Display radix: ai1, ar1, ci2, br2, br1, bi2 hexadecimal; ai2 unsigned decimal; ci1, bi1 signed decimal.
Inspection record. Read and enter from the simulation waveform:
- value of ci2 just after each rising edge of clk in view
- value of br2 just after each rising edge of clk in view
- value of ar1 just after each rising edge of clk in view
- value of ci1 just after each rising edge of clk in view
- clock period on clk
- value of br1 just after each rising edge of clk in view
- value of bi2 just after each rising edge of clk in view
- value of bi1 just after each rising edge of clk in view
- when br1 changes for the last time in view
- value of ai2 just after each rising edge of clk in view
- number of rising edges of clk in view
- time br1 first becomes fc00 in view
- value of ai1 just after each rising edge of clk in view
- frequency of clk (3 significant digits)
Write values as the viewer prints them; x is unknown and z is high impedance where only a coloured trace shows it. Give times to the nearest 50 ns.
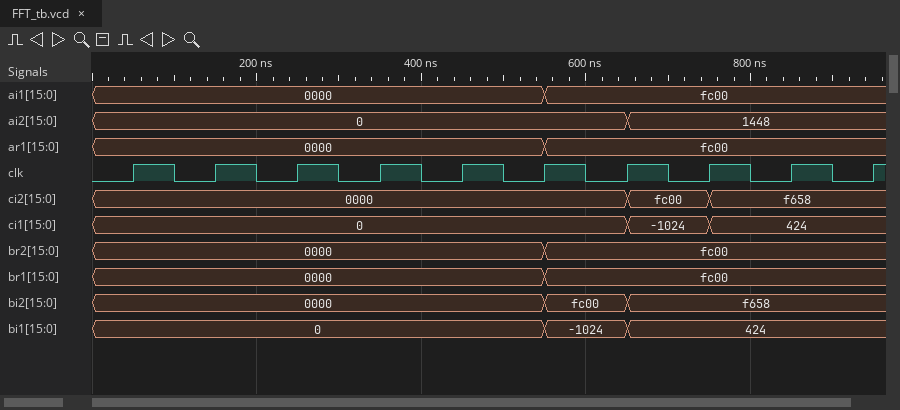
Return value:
0000, 0000, 0000, 0000, 0000, 0000, fc00, f658, f658, f658
0000, 0000, 0000, 0000, 0000, fc00, fc00, fc00, fc00, fc00
0000, 0000, 0000, 0000, 0000, fc00, fc00, fc00, fc00, fc00
0, 0, 0, 0, 0, 0, -1024, 424, 424, 424
100 ns
0000, 0000, 0000, 0000, 0000, fc00, fc00, fc00, fc00, fc00
0000, 0000, 0000, 0000, 0000, fc00, f658, f658, f658, f658
0, 0, 0, 0, 0, -1024, 424, 424, 424, 424
550 ns
0, 0, 0, 0, 0, 0, 1448, 1448, 1448, 1448
10
550 ns
0000, 0000, 0000, 0000, 0000, fc00, fc00, fc00, fc00, fc00
10.0 MHz
